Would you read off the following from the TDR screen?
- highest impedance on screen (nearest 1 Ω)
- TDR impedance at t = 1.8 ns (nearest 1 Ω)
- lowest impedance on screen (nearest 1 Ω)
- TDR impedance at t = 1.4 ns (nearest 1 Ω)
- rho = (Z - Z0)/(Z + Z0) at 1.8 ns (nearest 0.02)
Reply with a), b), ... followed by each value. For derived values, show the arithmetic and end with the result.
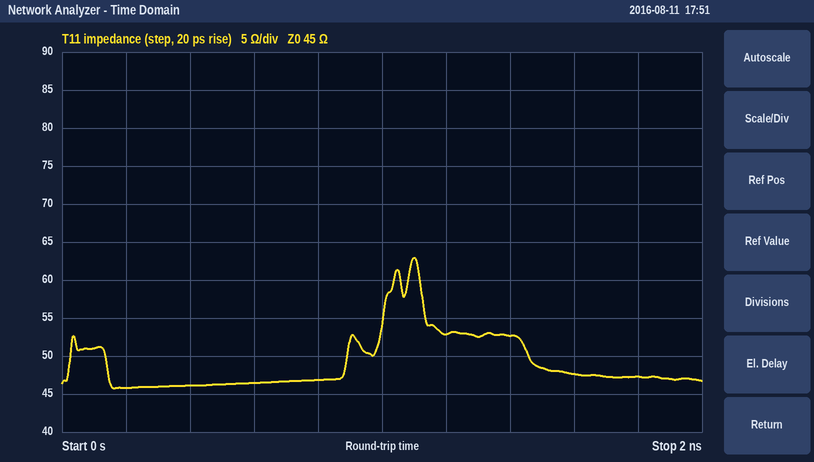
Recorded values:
a) 63 Ω
b) 47 Ω
c) 46 Ω
d) 53 Ω
e) (47 − 45)/(47 + 45) ≈ +0.02
